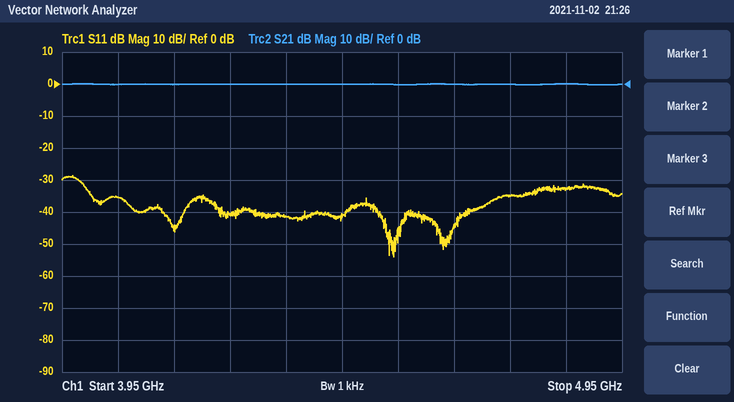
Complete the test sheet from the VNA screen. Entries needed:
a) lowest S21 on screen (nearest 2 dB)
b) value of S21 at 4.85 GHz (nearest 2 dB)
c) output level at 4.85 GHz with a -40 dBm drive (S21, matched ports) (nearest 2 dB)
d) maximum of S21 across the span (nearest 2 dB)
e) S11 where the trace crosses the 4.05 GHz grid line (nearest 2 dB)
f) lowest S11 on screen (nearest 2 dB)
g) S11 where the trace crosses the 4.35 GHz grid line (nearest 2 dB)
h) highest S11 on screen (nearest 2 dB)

0 dB
0 dB
-40 dBm
0 dB
-36 dB
-54 dB
-42 dB
-28 dB
